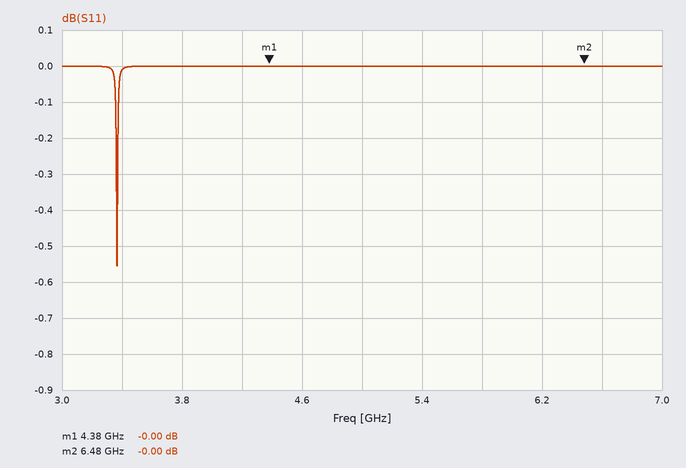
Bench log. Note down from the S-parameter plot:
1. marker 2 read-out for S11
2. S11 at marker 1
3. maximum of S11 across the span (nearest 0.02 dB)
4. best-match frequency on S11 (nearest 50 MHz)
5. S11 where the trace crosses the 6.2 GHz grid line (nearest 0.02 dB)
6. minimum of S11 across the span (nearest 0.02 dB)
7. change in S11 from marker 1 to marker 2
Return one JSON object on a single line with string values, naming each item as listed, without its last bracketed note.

{"marker 2 read-out for S11": "-0.00 dB", "S11 at marker 1": "-0.00 dB", "maximum of S11 across the span": "0.00 dB", "best-match frequency on S11": "3.35 GHz", "S11 where the trace crosses the 6.2 GHz grid line": "0.00 dB", "minimum of S11 across the span": "-0.56 dB", "change in S11 from marker 1 to marker 2": "0.00 dB"}
